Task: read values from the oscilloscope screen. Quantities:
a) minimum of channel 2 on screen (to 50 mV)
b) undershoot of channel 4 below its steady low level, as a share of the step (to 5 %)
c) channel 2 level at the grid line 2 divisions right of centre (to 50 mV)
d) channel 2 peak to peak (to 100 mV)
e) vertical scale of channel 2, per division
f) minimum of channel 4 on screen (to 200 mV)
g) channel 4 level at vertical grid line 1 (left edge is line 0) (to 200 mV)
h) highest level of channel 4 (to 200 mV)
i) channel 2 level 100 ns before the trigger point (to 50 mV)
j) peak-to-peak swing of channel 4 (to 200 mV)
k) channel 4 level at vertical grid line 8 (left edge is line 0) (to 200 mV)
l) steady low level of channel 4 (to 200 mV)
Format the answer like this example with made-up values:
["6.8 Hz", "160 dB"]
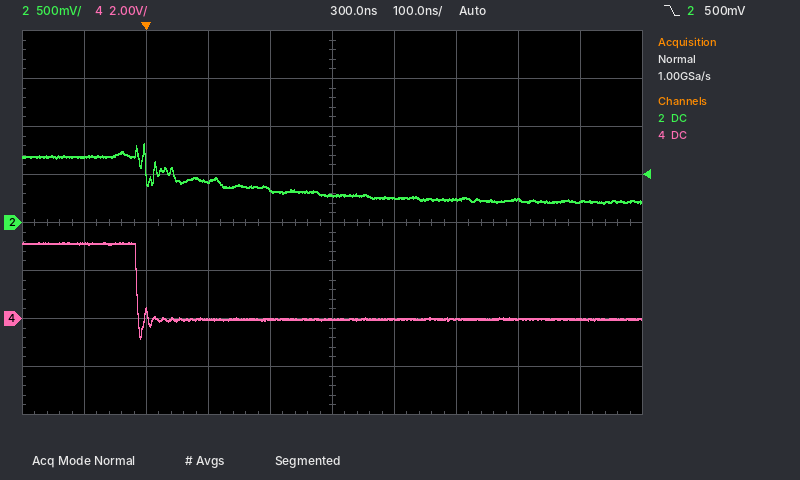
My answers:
["200 mV", "25 %", "250 mV", "600 mV", "500 mV", "-800 mV", "3.2 V", "3.2 V", "700 mV", "4.0 V", "0.0 V", "0.0 V"]
